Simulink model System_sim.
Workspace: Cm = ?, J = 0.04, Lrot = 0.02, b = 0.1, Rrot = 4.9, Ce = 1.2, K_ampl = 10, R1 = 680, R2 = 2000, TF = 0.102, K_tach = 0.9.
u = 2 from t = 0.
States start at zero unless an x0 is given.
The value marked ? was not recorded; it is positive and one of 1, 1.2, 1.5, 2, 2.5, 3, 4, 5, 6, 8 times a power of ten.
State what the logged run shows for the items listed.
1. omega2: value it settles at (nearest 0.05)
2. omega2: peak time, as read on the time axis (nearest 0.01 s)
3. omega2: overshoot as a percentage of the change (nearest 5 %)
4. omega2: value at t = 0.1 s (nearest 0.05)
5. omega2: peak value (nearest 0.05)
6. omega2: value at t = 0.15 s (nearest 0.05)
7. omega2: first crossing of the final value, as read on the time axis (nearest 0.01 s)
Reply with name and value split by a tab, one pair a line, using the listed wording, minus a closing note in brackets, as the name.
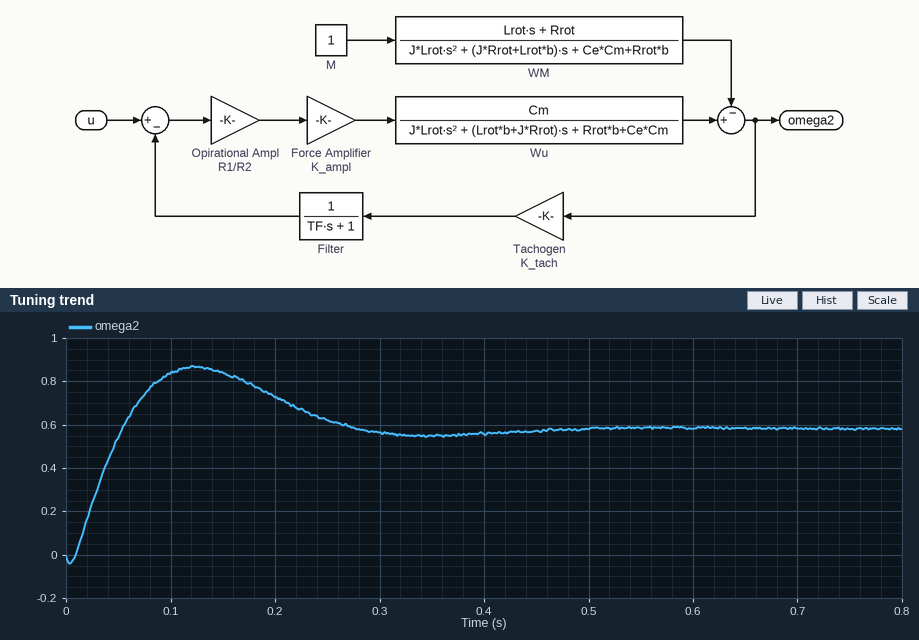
omega2: value it settles at	0.60
omega2: peak time, as read on the time axis	0.12 s
omega2: overshoot as a percentage of the change	50 %
omega2: value at t = 0.1 s	0.85
omega2: peak value	0.85
omega2: value at t = 0.15 s	0.85
omega2: first crossing of the final value, as read on the time axis	0.05 s
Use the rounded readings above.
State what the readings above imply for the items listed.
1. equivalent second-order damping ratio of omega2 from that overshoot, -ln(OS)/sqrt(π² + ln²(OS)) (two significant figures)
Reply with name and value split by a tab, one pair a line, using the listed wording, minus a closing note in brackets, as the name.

equivalent second-order damping ratio of omega2 from that overshoot, -ln(OS)/sqrt(π² + ln²(OS))	0.22
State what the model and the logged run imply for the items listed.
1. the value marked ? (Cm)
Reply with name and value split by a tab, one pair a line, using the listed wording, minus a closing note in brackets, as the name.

the value marked ?	1.2
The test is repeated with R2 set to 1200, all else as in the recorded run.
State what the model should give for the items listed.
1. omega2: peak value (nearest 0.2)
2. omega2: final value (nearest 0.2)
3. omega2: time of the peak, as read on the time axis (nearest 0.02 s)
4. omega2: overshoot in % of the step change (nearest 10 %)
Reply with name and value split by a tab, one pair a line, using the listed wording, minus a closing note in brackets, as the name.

omega2: peak value	2.0
omega2: final value	1.0
omega2: time of the peak, as read on the time axis	0.10 s
omega2: overshoot in % of the step change	80 %
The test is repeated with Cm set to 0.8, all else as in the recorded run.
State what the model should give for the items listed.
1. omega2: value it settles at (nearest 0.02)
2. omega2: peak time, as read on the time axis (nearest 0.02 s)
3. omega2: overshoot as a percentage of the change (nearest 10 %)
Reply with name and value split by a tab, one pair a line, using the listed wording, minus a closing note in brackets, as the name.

omega2: value it settles at	0.14
omega2: peak time, as read on the time axis	0.18 s
omega2: overshoot as a percentage of the change	40 %
